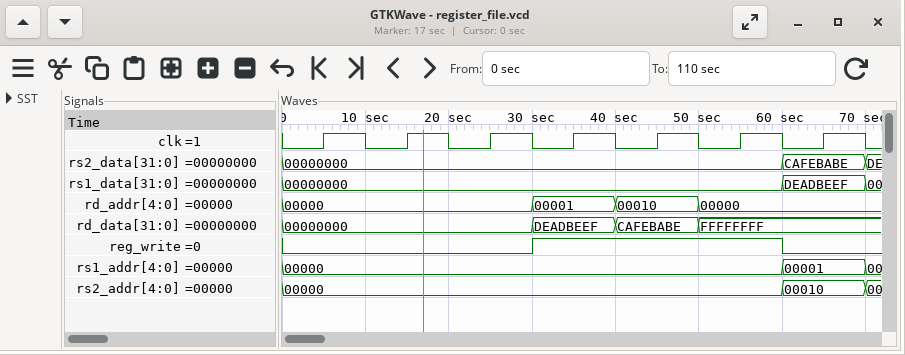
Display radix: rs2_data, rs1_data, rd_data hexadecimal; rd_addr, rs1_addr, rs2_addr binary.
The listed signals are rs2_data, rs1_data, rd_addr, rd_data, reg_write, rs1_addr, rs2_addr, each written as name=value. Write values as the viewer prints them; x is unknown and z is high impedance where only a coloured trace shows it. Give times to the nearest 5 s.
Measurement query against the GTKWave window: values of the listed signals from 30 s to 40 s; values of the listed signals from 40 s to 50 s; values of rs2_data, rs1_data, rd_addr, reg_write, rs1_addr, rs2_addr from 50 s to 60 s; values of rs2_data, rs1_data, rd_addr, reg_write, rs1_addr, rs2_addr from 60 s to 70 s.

rs2_data=00000000, rs1_data=00000000, rd_addr=00001, rd_data=DEADBEEF, reg_write=1, rs1_addr=00000, rs2_addr=00000
rs2_data=00000000, rs1_data=00000000, rd_addr=00010, rd_data=CAFEBABE, reg_write=1, rs1_addr=00000, rs2_addr=00000
rs2_data=00000000, rs1_data=00000000, rd_addr=00000, reg_write=1, rs1_addr=00000, rs2_addr=00000
rs2_data=CAFEBABE, rs1_data=DEADBEEF, rd_addr=00000, reg_write=0, rs1_addr=00001, rs2_addr=00010
